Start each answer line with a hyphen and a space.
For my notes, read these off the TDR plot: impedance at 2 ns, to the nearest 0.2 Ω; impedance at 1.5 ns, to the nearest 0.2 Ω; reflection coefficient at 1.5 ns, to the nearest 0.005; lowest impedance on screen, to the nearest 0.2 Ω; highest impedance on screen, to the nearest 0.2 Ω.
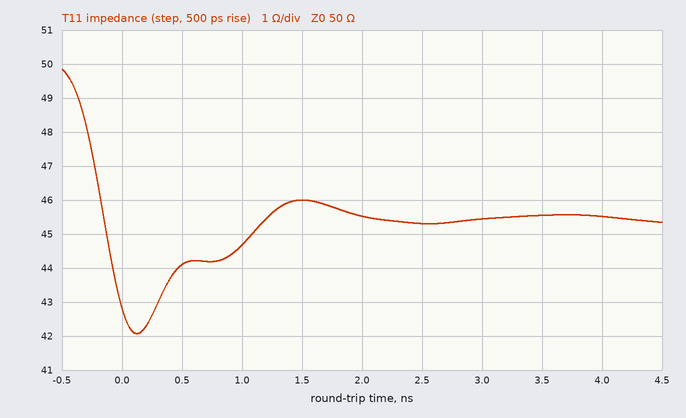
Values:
- 45.6 Ω
- 46.0 Ω
- -0.040
- 42.0 Ω
- 49.8 Ω
